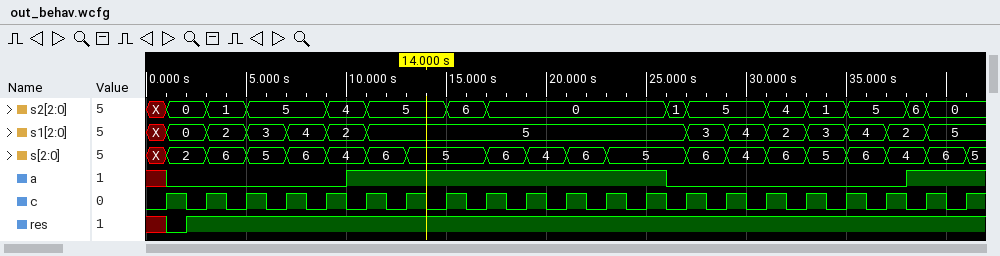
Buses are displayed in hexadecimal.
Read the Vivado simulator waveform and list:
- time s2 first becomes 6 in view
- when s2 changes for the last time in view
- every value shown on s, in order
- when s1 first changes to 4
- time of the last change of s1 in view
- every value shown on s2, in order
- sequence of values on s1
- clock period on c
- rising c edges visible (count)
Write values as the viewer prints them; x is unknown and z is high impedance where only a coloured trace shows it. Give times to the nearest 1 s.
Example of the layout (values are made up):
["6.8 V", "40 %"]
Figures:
["15 s", "39 s", "X, 2, 6, 5, 6, 4, 6, 5, 6, 4, 6, 5, 6, 4, 6, 5, 6, 4, 6, 5", "7 s", "39 s", "X, 0, 1, 5, 4, 5, 6, 0, 1, 5, 4, 1, 5, 6, 0", "X, 0, 2, 3, 4, 2, 5, 3, 4, 2, 3, 4, 2, 5", "2 s", "21"]
